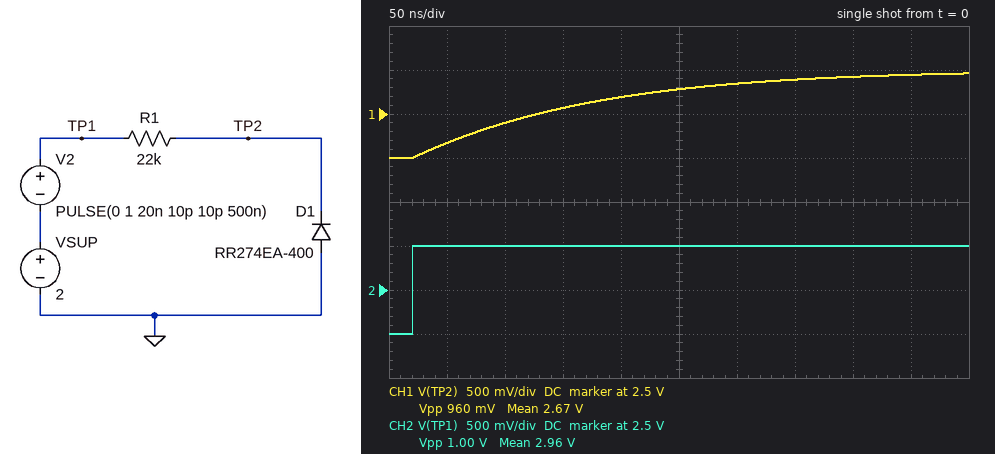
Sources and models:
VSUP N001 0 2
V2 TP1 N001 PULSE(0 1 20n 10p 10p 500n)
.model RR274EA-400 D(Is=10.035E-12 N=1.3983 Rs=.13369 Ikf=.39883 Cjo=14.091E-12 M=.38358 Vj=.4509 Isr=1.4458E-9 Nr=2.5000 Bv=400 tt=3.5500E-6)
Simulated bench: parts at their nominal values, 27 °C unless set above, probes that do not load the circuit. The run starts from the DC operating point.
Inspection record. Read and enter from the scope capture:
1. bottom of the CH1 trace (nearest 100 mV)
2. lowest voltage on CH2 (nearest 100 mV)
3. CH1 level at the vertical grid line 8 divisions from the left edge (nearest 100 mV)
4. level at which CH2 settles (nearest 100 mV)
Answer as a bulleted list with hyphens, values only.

- 2.0 V
- 2.0 V
- 2.9 V
- 3.0 V
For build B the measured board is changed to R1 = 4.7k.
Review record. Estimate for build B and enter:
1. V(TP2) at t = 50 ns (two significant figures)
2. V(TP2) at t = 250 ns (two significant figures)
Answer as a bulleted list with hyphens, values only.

- 2.6 V
- 3.0 V
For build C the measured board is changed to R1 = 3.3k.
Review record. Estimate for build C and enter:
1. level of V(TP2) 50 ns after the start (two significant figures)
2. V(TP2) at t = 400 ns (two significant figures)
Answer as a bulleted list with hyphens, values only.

- 2.7 V
- 3.0 V
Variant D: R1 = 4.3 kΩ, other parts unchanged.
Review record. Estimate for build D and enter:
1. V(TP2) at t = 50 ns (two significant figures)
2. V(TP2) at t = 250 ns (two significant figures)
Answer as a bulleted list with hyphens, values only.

- 2.6 V
- 3.0 V
